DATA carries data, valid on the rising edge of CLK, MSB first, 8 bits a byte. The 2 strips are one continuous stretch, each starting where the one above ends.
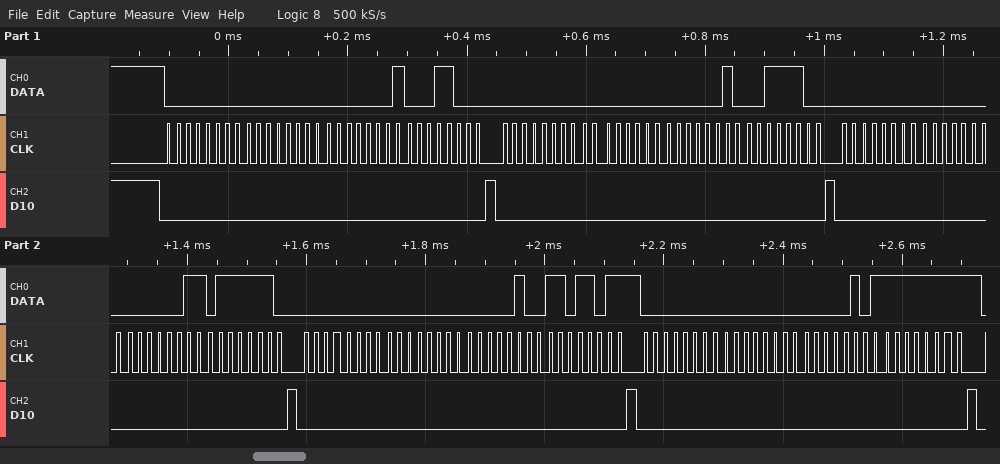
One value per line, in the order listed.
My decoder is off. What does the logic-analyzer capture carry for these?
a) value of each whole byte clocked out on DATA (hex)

00 00 01 18 00 00 02 3C 00 00 03 7E 00 00 04 DB 00 00 05 FF
